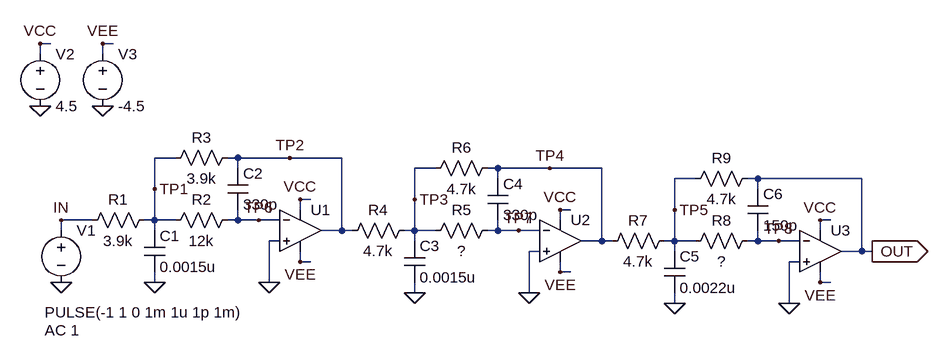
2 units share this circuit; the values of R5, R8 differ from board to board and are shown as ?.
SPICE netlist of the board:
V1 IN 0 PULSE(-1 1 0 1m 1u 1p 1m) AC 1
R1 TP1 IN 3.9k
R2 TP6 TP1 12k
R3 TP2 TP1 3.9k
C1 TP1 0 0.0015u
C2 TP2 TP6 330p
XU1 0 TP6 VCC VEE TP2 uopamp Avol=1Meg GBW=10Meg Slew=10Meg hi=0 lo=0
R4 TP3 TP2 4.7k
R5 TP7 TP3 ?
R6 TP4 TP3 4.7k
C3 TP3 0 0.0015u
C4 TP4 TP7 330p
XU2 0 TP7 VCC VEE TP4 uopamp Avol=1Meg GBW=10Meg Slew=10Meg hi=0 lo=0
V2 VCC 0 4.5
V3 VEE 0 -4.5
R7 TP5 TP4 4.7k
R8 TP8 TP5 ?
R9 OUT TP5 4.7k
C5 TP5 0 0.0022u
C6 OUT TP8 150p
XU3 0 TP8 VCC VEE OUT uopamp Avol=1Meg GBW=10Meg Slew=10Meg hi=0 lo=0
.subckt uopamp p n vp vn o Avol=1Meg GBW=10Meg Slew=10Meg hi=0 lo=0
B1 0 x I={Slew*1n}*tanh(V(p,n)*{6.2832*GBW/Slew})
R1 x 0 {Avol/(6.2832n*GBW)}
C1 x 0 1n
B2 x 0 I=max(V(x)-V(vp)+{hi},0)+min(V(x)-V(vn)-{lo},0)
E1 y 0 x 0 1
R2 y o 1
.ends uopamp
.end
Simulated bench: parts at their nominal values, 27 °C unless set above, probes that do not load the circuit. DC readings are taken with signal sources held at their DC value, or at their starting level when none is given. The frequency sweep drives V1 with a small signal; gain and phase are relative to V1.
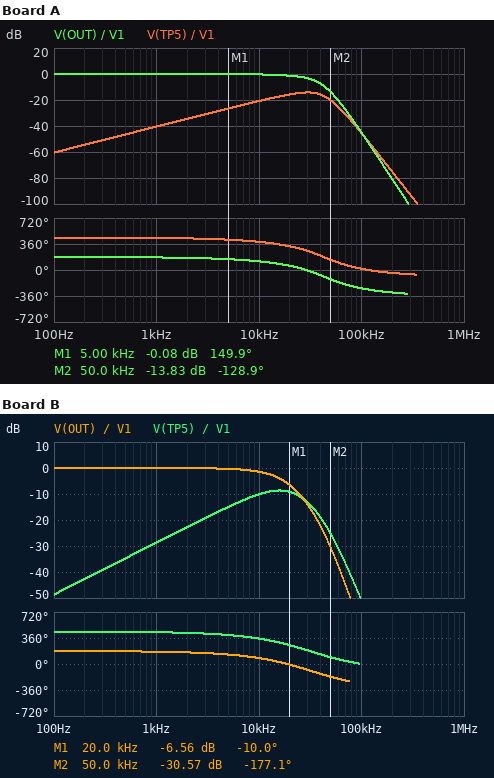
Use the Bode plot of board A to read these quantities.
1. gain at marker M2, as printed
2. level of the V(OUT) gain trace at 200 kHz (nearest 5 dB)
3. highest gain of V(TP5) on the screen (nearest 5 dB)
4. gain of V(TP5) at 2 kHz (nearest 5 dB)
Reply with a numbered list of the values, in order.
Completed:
1. -13.83 dB
2. -80 dB
3. -15 dB
4. -35 dB
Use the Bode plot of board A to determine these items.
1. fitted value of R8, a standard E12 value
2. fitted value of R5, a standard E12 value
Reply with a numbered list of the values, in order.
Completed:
1. 10 kΩ
2. 3.3 kΩ
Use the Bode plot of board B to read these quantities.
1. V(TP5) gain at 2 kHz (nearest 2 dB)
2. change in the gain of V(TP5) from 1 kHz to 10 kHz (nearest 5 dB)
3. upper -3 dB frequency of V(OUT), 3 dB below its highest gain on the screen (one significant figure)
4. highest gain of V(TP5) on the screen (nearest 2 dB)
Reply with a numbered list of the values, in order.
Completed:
1. -22 dB
2. 20 dB
3. 10 kHz
4. -8 dB
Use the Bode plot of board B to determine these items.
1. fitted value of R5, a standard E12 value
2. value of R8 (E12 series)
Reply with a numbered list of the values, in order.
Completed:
1. 5.6 kΩ
2. 39 kΩ
